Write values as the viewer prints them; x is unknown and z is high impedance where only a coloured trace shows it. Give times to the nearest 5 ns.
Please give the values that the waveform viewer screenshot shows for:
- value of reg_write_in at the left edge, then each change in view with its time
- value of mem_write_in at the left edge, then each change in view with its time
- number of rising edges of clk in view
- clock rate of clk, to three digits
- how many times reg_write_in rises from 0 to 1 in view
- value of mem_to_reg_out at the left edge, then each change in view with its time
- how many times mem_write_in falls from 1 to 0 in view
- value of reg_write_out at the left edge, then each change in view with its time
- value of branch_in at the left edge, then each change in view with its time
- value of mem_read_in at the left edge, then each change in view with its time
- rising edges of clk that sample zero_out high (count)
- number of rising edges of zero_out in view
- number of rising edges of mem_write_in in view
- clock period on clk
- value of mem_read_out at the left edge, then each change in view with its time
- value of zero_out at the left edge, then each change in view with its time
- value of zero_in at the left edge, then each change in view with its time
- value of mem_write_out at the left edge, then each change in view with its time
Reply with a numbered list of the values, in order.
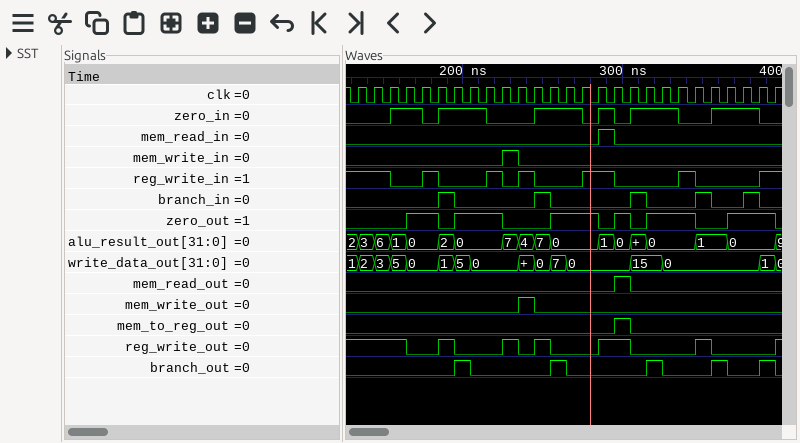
1. 1, 0 at 155 ns, 1 at 175 ns, 0 at 185 ns, 1 at 215 ns, 0 at 225 ns, 1 at 235 ns, 0 at 245 ns, 1 at 275 ns, 0 at 295 ns, 1 at 335 ns, 0 at 345 ns, 1 at 385 ns
2. 0, 1 at 225 ns, 0 at 235 ns
3. 27
4. 100 MHz
5. 6
6. 0, 1 at 295 ns, 0 at 305 ns
7. 1
8. 1, 0 at 165 ns, 1 at 185 ns, 0 at 195 ns, 1 at 225 ns, 0 at 235 ns, 1 at 245 ns, 0 at 255 ns, 1 at 285 ns, 0 at 305 ns, 1 at 345 ns, 0 at 355 ns, 1 at 395 ns
9. 0, 1 at 185 ns, 0 at 195 ns, 1 at 245 ns, 0 at 255 ns, 1 at 305 ns, 0 at 315 ns, 1 at 345 ns, 0 at 355 ns, 1 at 375 ns, 0 at 385 ns
10. 0, 1 at 285 ns, 0 at 295 ns
11. 15
12. 6
13. 1
14. 10 ns
15. 0, 1 at 295 ns, 0 at 305 ns
16. 0, 1 at 165 ns, 0 at 185 ns, 1 at 195 ns, 0 at 225 ns, 1 at 255 ns, 0 at 285 ns, 1 at 295 ns, 0 at 305 ns, 1 at 315 ns, 0 at 345 ns, 1 at 365 ns, 0 at 395 ns
17. 0, 1 at 155 ns, 0 at 175 ns, 1 at 185 ns, 0 at 215 ns, 1 at 245 ns, 0 at 275 ns, 1 at 285 ns, 0 at 295 ns, 1 at 305 ns, 0 at 335 ns, 1 at 355 ns, 0 at 385 ns
18. 0, 1 at 235 ns, 0 at 245 ns
